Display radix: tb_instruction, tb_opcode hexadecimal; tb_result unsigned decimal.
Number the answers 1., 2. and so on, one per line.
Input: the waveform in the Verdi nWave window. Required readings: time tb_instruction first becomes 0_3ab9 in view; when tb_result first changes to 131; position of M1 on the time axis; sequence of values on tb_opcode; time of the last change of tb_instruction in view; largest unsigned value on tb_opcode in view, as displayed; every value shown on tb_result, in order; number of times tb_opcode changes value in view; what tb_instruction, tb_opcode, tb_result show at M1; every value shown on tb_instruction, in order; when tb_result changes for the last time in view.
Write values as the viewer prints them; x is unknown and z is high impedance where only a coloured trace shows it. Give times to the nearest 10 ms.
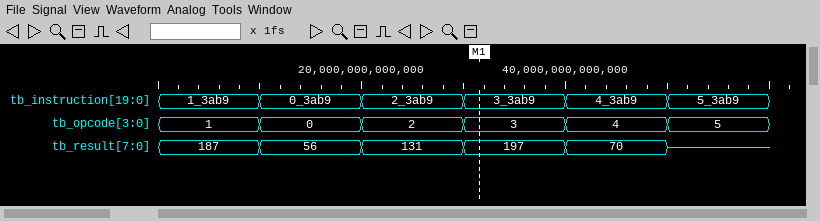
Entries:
1. 10 ms
2. 20 ms
3. 30 ms
4. 1, 0, 2, 3, 4, 5
5. 50 ms
6. 5
7. 187, 56, 131, 197, 70, z
8. 5
9. tb_instruction=3_3ab9, tb_opcode=3, tb_result=197
10. 1_3ab9, 0_3ab9, 2_3ab9, 3_3ab9, 4_3ab9, 5_3ab9
11. 50 ms
